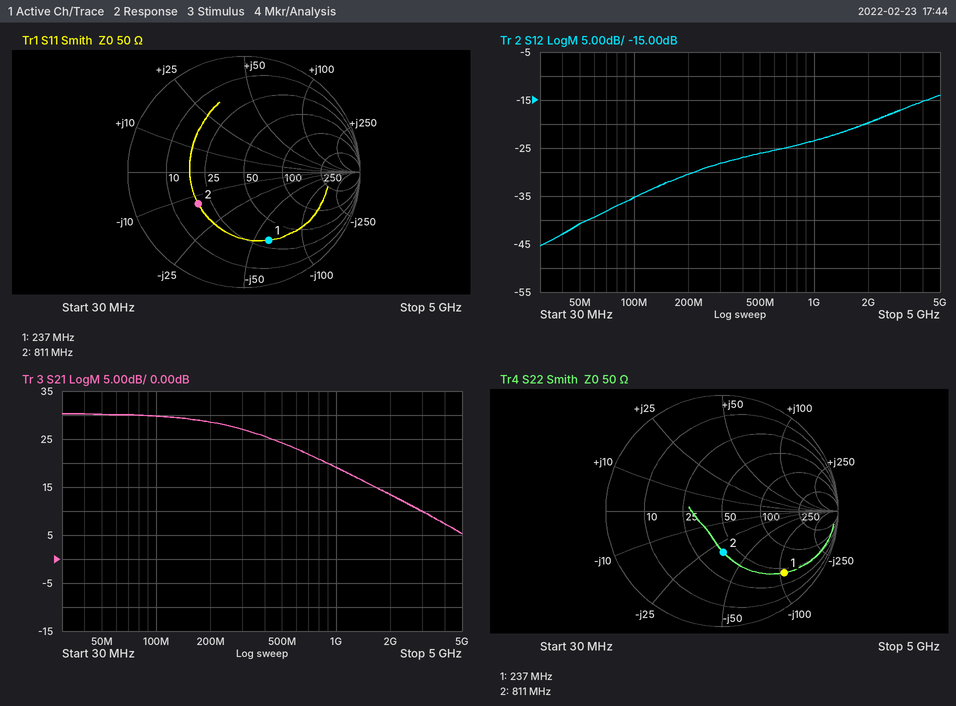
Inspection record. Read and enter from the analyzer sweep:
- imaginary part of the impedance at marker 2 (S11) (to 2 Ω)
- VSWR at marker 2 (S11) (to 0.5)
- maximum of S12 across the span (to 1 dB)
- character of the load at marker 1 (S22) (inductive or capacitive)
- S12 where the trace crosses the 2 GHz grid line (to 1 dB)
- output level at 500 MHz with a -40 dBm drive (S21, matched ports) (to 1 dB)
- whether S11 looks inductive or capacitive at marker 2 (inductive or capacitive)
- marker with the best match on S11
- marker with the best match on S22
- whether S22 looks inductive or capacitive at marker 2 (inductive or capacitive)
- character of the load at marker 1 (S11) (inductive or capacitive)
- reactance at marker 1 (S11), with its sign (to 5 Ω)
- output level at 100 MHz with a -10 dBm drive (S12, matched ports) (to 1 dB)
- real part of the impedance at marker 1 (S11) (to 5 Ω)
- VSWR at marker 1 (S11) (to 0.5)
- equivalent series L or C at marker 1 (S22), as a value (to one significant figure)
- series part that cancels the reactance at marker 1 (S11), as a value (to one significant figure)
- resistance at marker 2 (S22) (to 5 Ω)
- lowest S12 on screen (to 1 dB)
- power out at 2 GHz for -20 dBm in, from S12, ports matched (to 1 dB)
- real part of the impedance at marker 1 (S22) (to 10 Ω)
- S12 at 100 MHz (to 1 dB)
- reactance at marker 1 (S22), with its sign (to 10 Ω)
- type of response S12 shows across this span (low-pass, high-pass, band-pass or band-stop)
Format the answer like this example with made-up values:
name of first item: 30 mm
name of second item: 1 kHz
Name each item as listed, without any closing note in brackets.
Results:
imaginary part of the impedance at marker 2 (S11): -14 Ω
VSWR at marker 2 (S11): 3.0
maximum of S12 across the span: -14 dB
character of the load at marker 1 (S22): capacitive
S12 where the trace crosses the 2 GHz grid line: -20 dB
output level at 500 MHz with a -40 dBm drive (S21, matched ports): -16 dBm
whether S11 looks inductive or capacitive at marker 2: capacitive
marker with the best match on S11: marker 2
marker with the best match on S22: marker 2
whether S22 looks inductive or capacitive at marker 2: capacitive
character of the load at marker 1 (S11): capacitive
reactance at marker 1 (S11), with its sign: -60 Ω
output level at 100 MHz with a -10 dBm drive (S12, matched ports): -45 dBm
real part of the impedance at marker 1 (S11): 30 Ω
VSWR at marker 1 (S11): 4.5
equivalent series L or C at marker 1 (S22), as a value: 6 pF
series part that cancels the reactance at marker 1 (S11), as a value: 40 nH
resistance at marker 2 (S22): 40 Ω
lowest S12 on screen: -45 dB
power out at 2 GHz for -20 dBm in, from S12, ports matched: -40 dBm
real part of the impedance at marker 1 (S22): 40 Ω
S12 at 100 MHz: -35 dB
reactance at marker 1 (S22), with its sign: -110 Ω
type of response S12 shows across this span: high-pass
